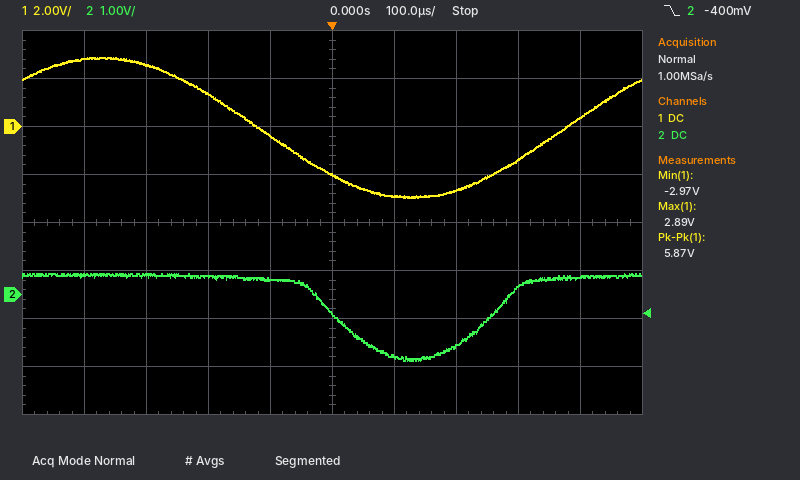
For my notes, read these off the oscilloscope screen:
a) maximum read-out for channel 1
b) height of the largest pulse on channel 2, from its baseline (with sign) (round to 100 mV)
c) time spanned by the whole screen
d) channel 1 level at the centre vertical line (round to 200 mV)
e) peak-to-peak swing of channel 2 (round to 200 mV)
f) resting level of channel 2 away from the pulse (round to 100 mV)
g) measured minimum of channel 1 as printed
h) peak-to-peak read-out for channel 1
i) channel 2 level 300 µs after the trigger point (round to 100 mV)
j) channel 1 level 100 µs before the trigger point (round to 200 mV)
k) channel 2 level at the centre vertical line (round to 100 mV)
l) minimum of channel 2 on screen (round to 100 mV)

2.89 V
-1.8 V
1 ms
-2.0 V
1.8 V
400 mV
-2.97 V
5.87 V
200 mV
-400 mV
-400 mV
-1.4 V
